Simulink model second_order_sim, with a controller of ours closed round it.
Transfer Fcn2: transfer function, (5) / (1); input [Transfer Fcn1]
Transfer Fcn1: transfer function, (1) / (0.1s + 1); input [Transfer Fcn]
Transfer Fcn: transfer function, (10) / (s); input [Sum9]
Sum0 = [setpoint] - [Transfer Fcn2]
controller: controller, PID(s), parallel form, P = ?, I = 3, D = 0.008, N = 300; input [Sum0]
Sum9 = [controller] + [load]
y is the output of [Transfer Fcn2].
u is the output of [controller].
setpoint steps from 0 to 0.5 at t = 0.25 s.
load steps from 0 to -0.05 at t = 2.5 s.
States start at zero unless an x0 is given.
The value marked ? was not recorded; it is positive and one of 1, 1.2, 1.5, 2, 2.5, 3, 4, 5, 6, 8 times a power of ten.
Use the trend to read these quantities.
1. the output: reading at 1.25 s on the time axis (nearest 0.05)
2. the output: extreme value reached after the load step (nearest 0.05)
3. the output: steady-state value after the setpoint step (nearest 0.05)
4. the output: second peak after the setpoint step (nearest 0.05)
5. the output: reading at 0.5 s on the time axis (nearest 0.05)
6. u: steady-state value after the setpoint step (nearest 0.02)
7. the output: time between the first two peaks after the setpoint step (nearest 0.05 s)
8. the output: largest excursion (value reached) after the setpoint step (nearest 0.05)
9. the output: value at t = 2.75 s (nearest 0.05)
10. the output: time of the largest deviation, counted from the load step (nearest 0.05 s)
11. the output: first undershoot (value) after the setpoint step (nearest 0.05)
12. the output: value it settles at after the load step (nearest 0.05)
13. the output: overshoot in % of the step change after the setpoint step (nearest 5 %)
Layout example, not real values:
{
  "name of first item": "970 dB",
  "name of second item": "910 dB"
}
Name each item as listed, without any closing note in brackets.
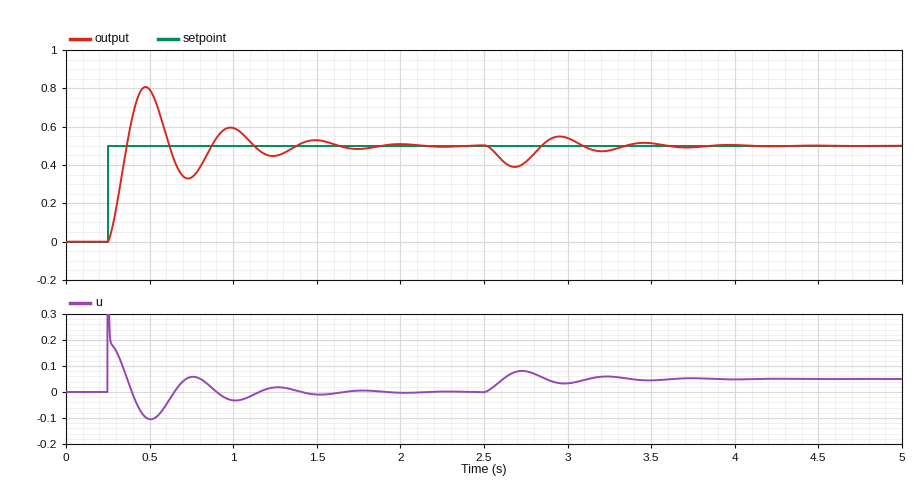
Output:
{
  "the output: reading at 1.25 s on the time axis": "0.45",
  "the output: extreme value reached after the load step": "0.40",
  "the output: steady-state value after the setpoint step": "0.50",
  "the output: second peak after the setpoint step": "0.60",
  "the output: reading at 0.5 s on the time axis": "0.80",
  "u: steady-state value after the setpoint step": "0.00",
  "the output: time between the first two peaks after the setpoint step": "0.50 s",
  "the output: largest excursion (value reached) after the setpoint step": "0.80",
  "the output: value at t = 2.75 s": "0.40",
  "the output: time of the largest deviation, counted from the load step": "0.20 s",
  "the output: first undershoot (value) after the setpoint step": "0.35",
  "the output: value it settles at after the load step": "0.50",
  "the output: overshoot in % of the step change after the setpoint step": "60 %"
}
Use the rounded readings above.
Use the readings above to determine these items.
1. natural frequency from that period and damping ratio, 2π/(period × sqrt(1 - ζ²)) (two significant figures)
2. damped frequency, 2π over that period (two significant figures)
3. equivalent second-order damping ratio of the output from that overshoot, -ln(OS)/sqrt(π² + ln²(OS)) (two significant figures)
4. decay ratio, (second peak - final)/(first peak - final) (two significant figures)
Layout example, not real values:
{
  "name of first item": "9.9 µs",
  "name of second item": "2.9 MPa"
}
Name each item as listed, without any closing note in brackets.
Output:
{
  "natural frequency from that period and damping ratio, 2π/(period × sqrt(1 - ζ²))": "13 rad/s",
  "damped frequency, 2π over that period": "13 rad/s",
  "equivalent second-order damping ratio of the output from that overshoot, -ln(OS)/sqrt(π² + ln²(OS))": "0.16",
  "decay ratio, (second peak - final)/(first peak - final)": "0.33"
}
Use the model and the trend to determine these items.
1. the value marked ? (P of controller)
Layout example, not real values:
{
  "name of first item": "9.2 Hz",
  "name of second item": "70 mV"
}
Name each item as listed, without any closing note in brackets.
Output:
{
  "the value marked ?": "0.4"
}
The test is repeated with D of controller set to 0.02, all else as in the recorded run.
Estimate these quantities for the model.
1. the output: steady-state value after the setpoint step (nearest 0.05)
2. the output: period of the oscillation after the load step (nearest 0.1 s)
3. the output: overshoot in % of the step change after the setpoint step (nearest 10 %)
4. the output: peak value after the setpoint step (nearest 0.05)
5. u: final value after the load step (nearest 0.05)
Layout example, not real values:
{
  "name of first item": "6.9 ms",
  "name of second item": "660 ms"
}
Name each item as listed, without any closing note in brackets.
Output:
{
  "the output: steady-state value after the setpoint step": "0.50",
  "the output: period of the oscillation after the load step": "0.6 s",
  "the output: overshoot in % of the step change after the setpoint step": "40 %",
  "the output: peak value after the setpoint step": "0.70",
  "u: final value after the load step": "0.05"
}
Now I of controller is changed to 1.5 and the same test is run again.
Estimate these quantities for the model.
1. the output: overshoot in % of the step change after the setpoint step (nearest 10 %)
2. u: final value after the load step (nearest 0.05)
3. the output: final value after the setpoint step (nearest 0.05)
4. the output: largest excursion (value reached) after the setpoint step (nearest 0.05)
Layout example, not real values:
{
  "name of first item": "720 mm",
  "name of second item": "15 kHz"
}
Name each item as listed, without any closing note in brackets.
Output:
{
  "the output: overshoot in % of the step change after the setpoint step": "40 %",
  "u: final value after the load step": "0.05",
  "the output: final value after the setpoint step": "0.50",
  "the output: largest excursion (value reached) after the setpoint step": "0.70"
}
